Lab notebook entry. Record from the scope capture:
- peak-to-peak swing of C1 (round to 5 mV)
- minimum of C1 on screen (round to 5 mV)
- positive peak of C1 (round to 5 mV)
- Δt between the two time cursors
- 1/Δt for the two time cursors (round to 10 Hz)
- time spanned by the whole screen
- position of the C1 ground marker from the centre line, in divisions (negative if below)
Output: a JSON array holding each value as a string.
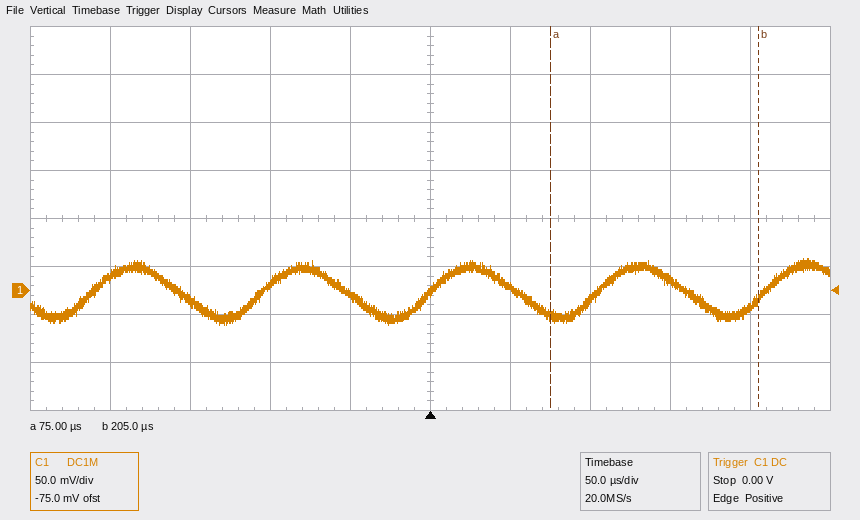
["70 mV", "-35 mV", "35 mV", "130 µs", "7.69 kHz", "500 µs", "-1.5 div"]
